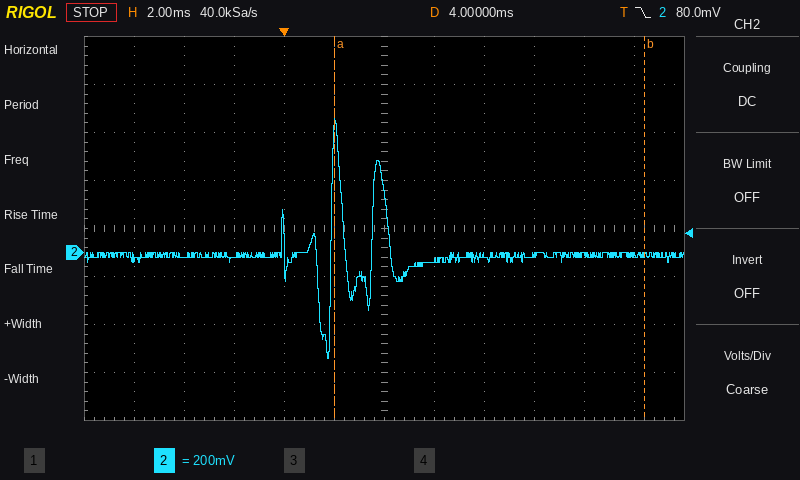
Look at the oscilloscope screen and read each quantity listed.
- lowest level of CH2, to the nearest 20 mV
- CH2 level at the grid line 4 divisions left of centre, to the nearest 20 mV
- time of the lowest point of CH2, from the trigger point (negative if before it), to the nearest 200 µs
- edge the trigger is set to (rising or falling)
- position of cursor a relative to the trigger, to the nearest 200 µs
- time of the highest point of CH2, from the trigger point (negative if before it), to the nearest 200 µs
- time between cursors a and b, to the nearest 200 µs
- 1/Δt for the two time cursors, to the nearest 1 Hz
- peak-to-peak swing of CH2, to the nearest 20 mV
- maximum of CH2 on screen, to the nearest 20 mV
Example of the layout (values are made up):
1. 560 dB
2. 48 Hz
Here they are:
1. -440 mV
2. -20 mV
3. +1.8 ms
4. falling
5. +2.0 ms
6. +2.0 ms
7. 12.4 ms
8. 81 Hz
9. 1.00 V
10. 560 mV
